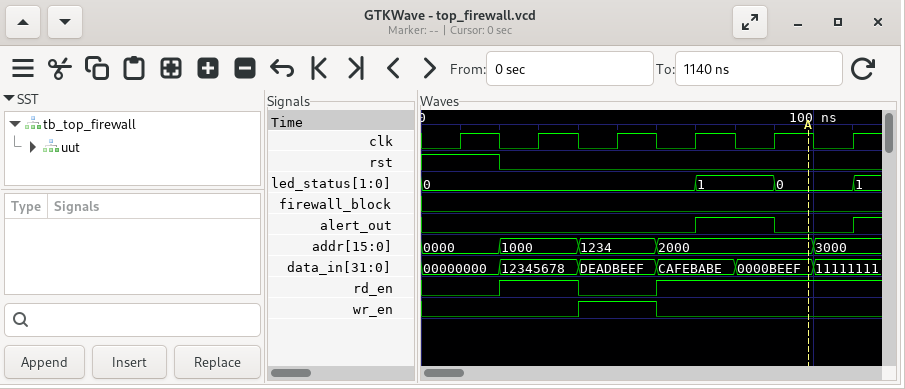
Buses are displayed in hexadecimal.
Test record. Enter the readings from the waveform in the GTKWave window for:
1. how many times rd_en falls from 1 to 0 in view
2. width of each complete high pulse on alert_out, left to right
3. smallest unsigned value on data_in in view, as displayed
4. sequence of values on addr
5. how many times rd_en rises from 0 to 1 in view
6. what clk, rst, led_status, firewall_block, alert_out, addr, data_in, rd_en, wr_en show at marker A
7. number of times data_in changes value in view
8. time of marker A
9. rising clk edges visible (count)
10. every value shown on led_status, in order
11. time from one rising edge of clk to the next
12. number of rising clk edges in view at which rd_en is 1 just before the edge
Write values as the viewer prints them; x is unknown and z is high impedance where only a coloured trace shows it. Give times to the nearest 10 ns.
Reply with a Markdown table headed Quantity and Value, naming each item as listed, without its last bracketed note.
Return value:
| Quantity | Value |
|---|---|
| how many times rd_en falls from 1 to 0 in view | 1 |
| width of each complete high pulse on alert_out, left to right | 20 ns |
| smallest unsigned value on data_in in view, as displayed | 00000000 |
| sequence of values on addr | 0000, 1000, 1234, 2000, 3000 |
| how many times rd_en rises from 0 to 1 in view | 2 |
| what clk, rst, led_status, firewall_block, alert_out, addr, data_in, rd_en, wr_en show at marker A | clk=1, rst=0, led_status=0, firewall_block=0, alert_out=0, addr=2000, data_in=0000BEEF, rd_en=1, wr_en=0 |
| number of times data_in changes value in view | 5 |
| time of marker A | 100 ns |
| rising clk edges visible | 6 |
| every value shown on led_status, in order | 0, 1, 0, 1 |
| time from one rising edge of clk to the next | 20 ns |
| number of rising clk edges in view at which rd_en is 1 just before the edge | 4 |
